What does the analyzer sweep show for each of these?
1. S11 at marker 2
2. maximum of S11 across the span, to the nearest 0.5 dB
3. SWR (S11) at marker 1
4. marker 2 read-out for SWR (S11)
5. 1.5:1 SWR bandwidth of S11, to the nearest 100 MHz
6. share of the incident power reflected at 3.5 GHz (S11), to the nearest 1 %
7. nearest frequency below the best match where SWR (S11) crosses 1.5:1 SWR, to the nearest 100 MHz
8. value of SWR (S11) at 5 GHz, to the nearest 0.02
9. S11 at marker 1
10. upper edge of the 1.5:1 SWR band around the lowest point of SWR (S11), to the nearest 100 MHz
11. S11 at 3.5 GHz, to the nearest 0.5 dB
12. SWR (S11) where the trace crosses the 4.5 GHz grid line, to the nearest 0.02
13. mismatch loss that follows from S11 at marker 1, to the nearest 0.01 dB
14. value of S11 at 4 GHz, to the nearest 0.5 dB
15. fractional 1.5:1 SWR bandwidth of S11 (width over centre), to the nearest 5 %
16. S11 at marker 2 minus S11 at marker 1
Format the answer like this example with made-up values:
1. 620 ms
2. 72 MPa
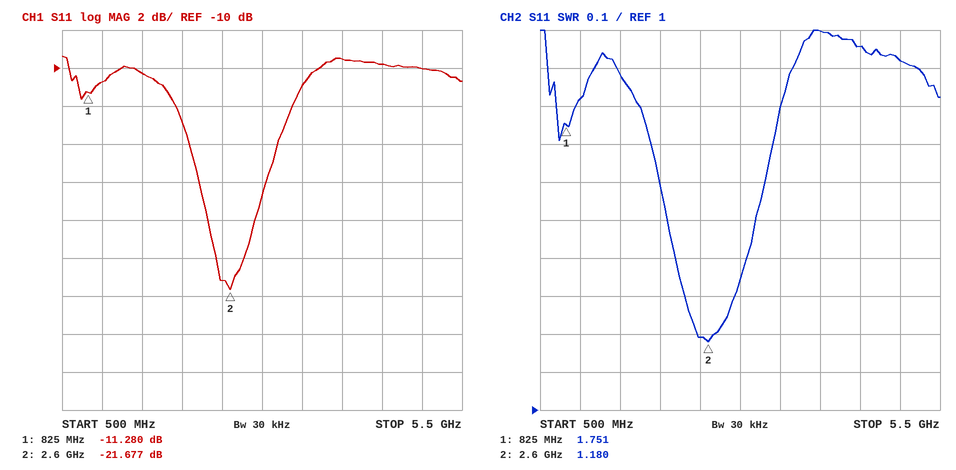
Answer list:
1. -21.677 dB
2. -9.5 dB
3. 1.751
4. 1.180
5. 1.1 GHz
6. 8 %
7. 2.1 GHz
8. 1.92
9. -11.280 dB
10. 3.2 GHz
11. -11.0 dB
12. 1.96
13. 0.34 dB
14. -9.5 dB
15. 40 %
16. -10.397 dB
